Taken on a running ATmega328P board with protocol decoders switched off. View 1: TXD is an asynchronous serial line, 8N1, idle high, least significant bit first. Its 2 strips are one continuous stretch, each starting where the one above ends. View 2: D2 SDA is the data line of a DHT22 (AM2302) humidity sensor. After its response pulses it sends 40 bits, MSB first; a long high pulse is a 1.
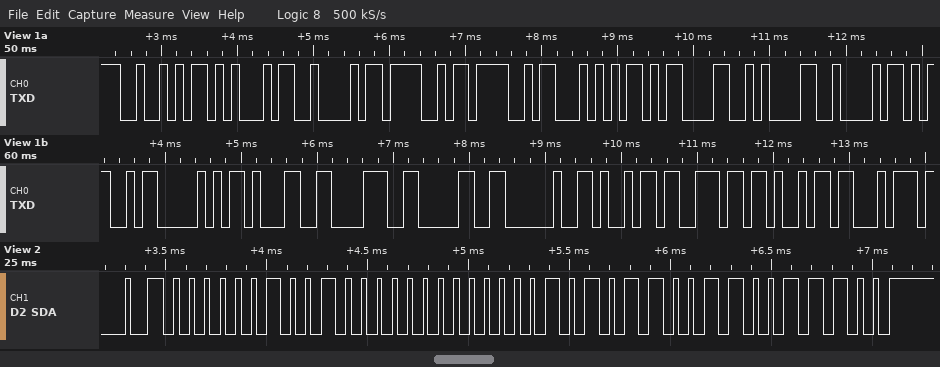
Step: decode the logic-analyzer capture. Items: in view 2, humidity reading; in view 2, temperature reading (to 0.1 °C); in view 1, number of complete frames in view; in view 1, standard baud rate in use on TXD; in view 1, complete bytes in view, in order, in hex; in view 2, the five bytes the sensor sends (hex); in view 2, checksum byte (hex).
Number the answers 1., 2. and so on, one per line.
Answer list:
1. 57.6 %
2. 34.5 °C
3. 19
4. 9600 baud
5. 52 45 42 4F 4F 54 0D 0A 42 4D 50 31 38 30 20 69 6E 69 74
6. 02 40 01 59 9C
7. 0x9C
